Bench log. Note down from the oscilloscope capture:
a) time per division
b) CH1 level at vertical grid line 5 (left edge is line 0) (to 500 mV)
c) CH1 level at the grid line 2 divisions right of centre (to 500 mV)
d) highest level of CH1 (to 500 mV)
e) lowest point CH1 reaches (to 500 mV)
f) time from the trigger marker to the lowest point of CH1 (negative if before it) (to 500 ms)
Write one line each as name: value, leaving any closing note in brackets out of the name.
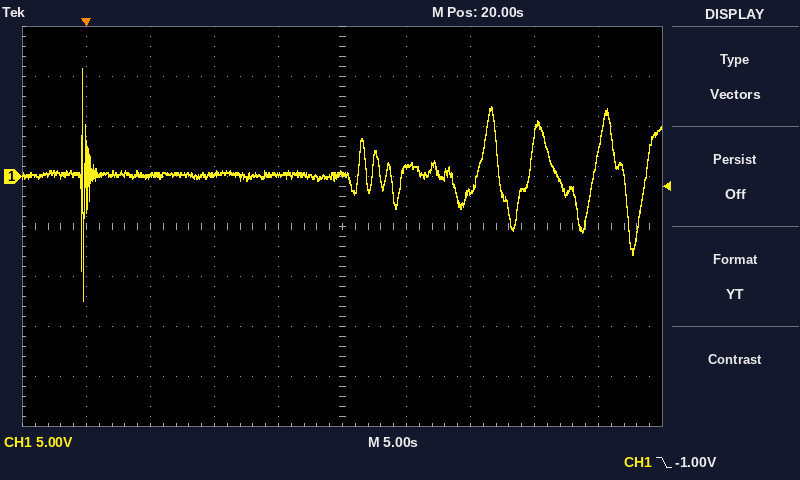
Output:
time per division: 5 s
CH1 level at vertical grid line 5 (left edge is line 0): 500 mV
CH1 level at the grid line 2 divisions right of centre: -1.5 V
highest level of CH1: 11.0 V
lowest point CH1 reaches: -12.5 V
time from the trigger marker to the lowest point of CH1 (negative if before it): 0.0 s
